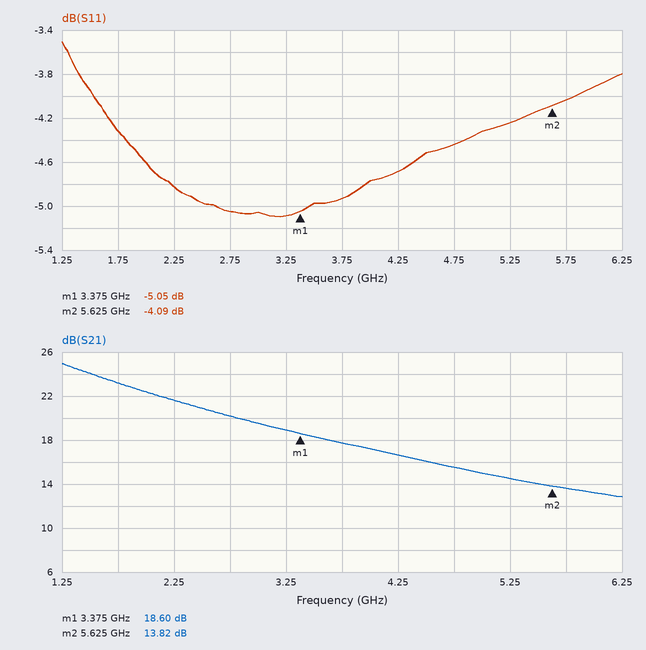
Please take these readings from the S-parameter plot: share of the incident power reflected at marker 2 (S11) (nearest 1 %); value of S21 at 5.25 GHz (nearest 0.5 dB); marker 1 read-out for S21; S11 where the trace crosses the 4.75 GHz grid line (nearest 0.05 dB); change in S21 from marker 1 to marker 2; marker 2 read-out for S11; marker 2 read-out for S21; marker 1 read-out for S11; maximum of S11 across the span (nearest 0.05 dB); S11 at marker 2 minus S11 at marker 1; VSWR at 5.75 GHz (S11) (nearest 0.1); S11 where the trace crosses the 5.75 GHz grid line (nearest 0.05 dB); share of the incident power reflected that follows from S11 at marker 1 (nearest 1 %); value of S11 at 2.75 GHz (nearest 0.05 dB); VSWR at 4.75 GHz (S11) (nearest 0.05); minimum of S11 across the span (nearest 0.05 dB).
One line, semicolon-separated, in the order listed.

39 %; 14.5 dB; 18.60 dB; -4.45 dB; -4.78 dB; -4.09 dB; 13.82 dB; -5.05 dB; -3.50 dB; 0.96 dB; 4.4; -4.05 dB; 31 %; -5.05 dB; 4.00; -5.10 dB
